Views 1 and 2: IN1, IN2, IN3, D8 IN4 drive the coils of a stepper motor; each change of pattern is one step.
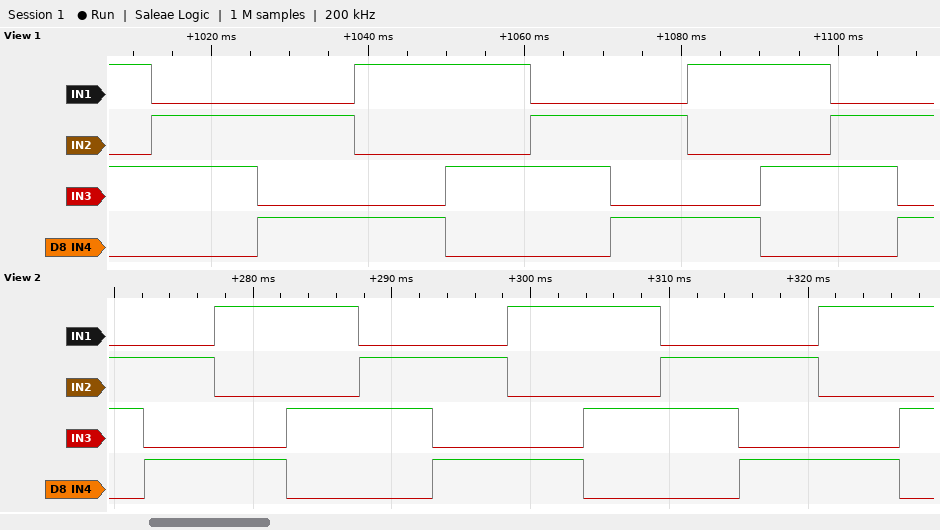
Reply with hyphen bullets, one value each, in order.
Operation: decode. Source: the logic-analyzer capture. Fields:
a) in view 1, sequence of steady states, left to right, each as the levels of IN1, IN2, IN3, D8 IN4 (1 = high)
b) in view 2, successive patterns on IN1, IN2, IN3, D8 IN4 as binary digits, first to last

- 1010 0110 0101 1001 1010 0110 0101 1001 1010 0110 0101
- 0110 0101 1001 1010 0110 0101 1001 1010 0110 0101 1001 1010
